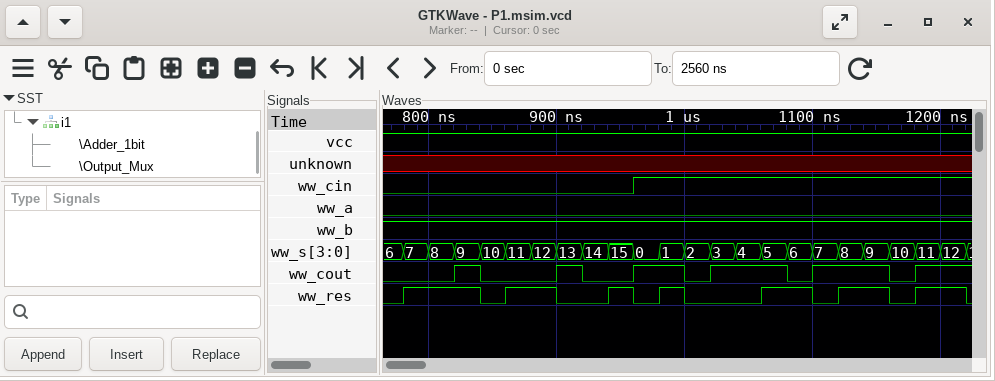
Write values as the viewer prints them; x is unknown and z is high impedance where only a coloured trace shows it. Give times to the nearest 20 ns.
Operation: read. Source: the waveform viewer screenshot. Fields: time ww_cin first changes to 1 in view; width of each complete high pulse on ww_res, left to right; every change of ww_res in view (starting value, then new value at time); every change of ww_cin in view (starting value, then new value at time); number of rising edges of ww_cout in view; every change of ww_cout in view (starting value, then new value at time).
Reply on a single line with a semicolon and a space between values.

960 ns; 60 ns, 40 ns, 20 ns, 20 ns, 40 ns, 40 ns, 40 ns; 0, 1 at 780 ns, 0 at 840 ns, 1 at 860 ns, 0 at 900 ns, 1 at 940 ns, 0 at 960 ns, 1 at 980 ns, 0 at 1000 ns, 1 at 1060 ns, 0 at 1100 ns, 1 at 1120 ns, 0 at 1160 ns, 1 at 1180 ns, 0 at 1220 ns; 0, 1 at 960 ns; 6; 0, 1 at 820 ns, 0 at 840 ns, 1 at 900 ns, 0 at 920 ns, 1 at 960 ns, 0 at 1000 ns, 1 at 1020 ns, 0 at 1080 ns, 1 at 1100 ns, 0 at 1160 ns, 1 at 1180 ns
